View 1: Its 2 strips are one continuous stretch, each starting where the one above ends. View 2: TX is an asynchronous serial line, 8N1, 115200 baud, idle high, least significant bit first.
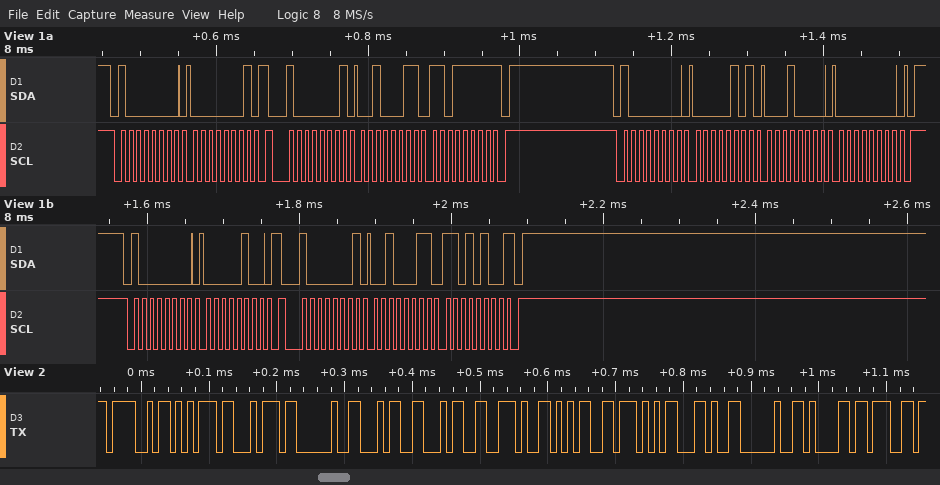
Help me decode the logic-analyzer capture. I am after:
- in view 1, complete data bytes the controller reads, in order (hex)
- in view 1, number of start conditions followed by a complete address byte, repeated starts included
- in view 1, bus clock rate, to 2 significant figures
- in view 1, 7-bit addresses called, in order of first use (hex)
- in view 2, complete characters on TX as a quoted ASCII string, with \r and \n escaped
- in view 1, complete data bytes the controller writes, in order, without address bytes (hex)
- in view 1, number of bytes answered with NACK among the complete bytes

23 DF 23 D4
5
100 kHz
0x40
"Out 44.5W, ag"
01 05 10 00 04
2
